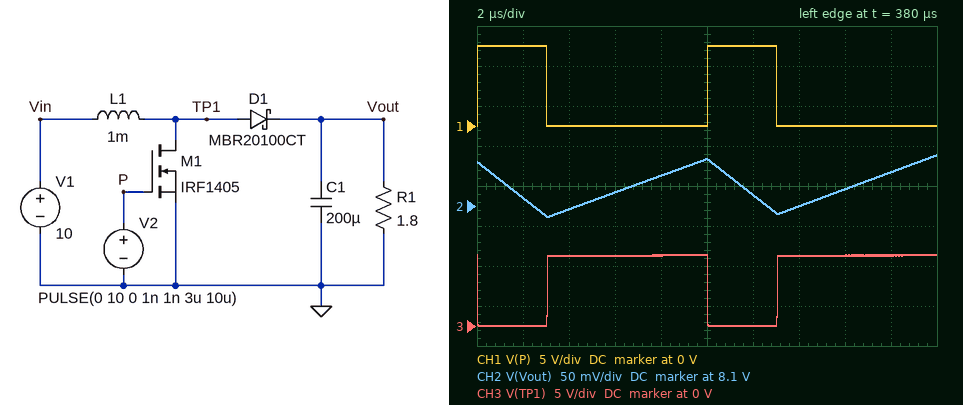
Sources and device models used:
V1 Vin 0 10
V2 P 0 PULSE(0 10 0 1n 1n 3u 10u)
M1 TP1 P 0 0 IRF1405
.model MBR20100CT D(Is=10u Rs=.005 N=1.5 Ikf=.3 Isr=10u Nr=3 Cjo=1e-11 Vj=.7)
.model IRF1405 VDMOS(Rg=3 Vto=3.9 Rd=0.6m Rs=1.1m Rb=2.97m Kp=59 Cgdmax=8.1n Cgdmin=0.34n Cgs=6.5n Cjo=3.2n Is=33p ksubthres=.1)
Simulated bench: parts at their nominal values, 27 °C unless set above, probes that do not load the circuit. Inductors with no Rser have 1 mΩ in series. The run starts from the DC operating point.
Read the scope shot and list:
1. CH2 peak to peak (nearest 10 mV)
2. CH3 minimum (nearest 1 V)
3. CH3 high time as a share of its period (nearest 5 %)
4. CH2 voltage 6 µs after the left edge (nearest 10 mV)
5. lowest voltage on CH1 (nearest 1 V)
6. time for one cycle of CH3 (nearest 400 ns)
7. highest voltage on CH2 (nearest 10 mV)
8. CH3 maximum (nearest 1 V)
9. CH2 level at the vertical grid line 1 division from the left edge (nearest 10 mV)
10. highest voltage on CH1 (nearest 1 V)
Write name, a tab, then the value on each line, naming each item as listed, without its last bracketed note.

CH2 peak to peak	80 mV
CH3 minimum	0 V
CH3 high time as a share of its period	70 %
CH2 voltage 6 µs after the left edge	8.12 V
lowest voltage on CH1	0 V
time for one cycle of CH3	10.0 µs
highest voltage on CH2	8.16 V
CH3 maximum	9 V
CH2 level at the vertical grid line 1 division from the left edge	8.11 V
highest voltage on CH1	10 V
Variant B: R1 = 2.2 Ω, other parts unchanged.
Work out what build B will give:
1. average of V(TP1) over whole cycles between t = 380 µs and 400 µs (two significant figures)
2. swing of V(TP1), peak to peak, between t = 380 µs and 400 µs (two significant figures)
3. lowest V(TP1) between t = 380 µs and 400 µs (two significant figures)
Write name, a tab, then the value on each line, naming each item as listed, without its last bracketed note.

average of V(TP1) over whole cycles between t = 380 µs and 400 µs	6.3 V
swing of V(TP1), peak to peak, between t = 380 µs and 400 µs	9.1 V
lowest V(TP1) between t = 380 µs and 400 µs	17 mV
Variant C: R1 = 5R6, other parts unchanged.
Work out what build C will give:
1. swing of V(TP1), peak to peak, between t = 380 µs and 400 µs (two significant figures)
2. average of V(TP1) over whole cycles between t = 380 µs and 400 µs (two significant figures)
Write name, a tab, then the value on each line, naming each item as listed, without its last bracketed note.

swing of V(TP1), peak to peak, between t = 380 µs and 400 µs	10 V
average of V(TP1) over whole cycles between t = 380 µs and 400 µs	6.9 V
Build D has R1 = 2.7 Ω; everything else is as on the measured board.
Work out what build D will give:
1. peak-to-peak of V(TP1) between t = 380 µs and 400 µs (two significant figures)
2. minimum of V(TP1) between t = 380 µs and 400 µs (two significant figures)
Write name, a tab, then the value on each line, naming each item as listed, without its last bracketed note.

peak-to-peak of V(TP1) between t = 380 µs and 400 µs	9.3 V
minimum of V(TP1) between t = 380 µs and 400 µs	13 mV
